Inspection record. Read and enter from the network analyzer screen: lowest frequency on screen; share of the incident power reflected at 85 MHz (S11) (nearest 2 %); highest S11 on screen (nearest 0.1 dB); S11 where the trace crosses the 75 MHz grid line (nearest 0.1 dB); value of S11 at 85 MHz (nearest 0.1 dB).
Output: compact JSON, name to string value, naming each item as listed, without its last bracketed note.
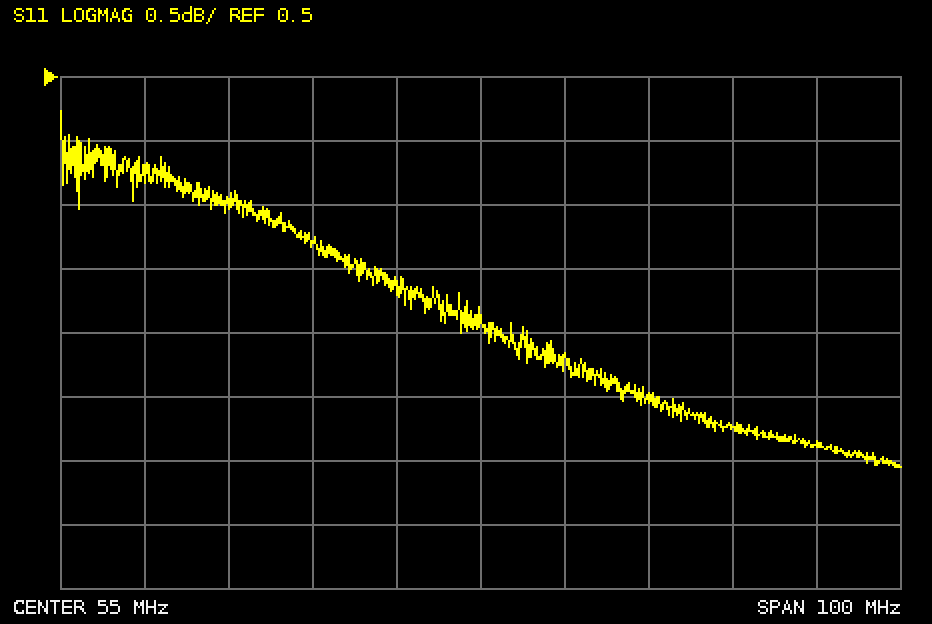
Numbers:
{"lowest frequency on screen": "5 MHz", "share of the incident power reflected at 85 MHz (S11)": "60 %", "highest S11 on screen": "0.2 dB", "S11 where the trace crosses the 75 MHz grid line": "-2.0 dB", "value of S11 at 85 MHz": "-2.2 dB"}
